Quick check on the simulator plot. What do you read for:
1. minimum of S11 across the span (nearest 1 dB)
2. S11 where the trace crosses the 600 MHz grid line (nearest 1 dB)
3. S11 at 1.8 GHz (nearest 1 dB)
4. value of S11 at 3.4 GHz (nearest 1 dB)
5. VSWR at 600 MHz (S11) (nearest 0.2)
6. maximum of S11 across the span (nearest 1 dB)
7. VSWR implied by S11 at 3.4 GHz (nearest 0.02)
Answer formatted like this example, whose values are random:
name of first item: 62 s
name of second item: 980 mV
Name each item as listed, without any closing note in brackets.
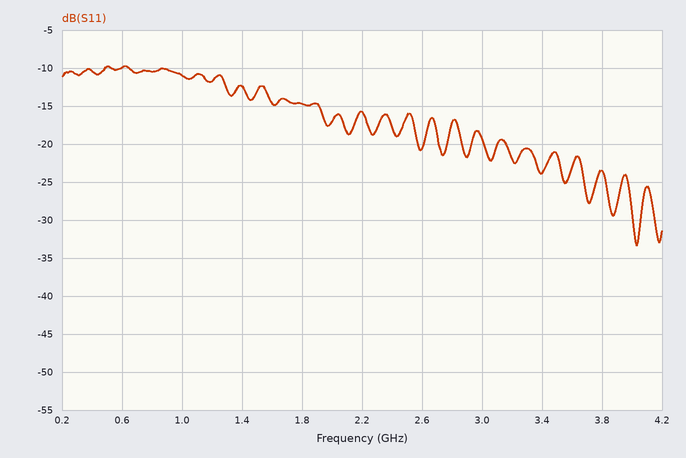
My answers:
minimum of S11 across the span: -33 dB
S11 where the trace crosses the 600 MHz grid line: -10 dB
S11 at 1.8 GHz: -15 dB
value of S11 at 3.4 GHz: -24 dB
VSWR at 600 MHz (S11): 2.0
maximum of S11 across the span: -10 dB
VSWR implied by S11 at 3.4 GHz: 1.14
